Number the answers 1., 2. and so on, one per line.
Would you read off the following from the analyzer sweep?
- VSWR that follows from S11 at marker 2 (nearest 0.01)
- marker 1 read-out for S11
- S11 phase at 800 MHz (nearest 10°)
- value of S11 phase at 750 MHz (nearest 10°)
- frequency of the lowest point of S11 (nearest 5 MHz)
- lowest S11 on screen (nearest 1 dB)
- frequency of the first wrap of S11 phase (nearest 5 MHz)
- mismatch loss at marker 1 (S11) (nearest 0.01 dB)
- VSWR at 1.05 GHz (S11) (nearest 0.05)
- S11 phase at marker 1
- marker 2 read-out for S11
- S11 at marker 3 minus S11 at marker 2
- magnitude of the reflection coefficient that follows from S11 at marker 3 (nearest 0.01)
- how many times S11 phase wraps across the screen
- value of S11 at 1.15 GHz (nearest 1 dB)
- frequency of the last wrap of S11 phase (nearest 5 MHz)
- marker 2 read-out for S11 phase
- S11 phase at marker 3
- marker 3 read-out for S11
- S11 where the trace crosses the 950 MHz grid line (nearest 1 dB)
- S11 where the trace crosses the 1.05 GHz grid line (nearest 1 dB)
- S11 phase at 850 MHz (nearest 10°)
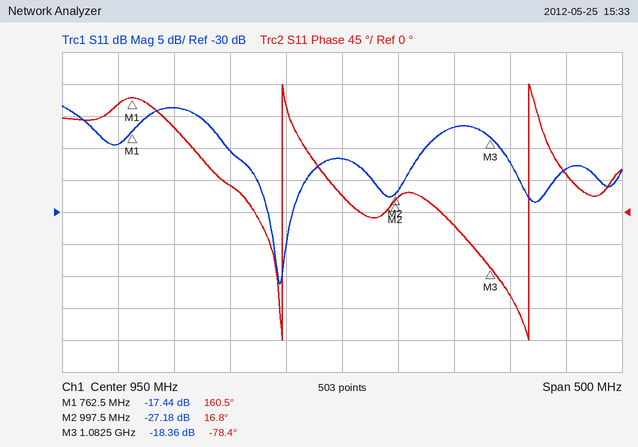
1. 1.09
2. -17.44 dB
3. 120°
4. 150°
5. 895 MHz
6. -41 dB
7. 895 MHz
8. 0.08 dB
9. 1.35
10. 160.5°
11. -27.18 dB
12. 8.82 dB
13. 0.12
14. 2
15. -23 dB
16. 1.115 GHz
17. 16.8°
18. -78.4°
19. -18.36 dB
20. -22 dB
21. -17 dB
22. 40°
